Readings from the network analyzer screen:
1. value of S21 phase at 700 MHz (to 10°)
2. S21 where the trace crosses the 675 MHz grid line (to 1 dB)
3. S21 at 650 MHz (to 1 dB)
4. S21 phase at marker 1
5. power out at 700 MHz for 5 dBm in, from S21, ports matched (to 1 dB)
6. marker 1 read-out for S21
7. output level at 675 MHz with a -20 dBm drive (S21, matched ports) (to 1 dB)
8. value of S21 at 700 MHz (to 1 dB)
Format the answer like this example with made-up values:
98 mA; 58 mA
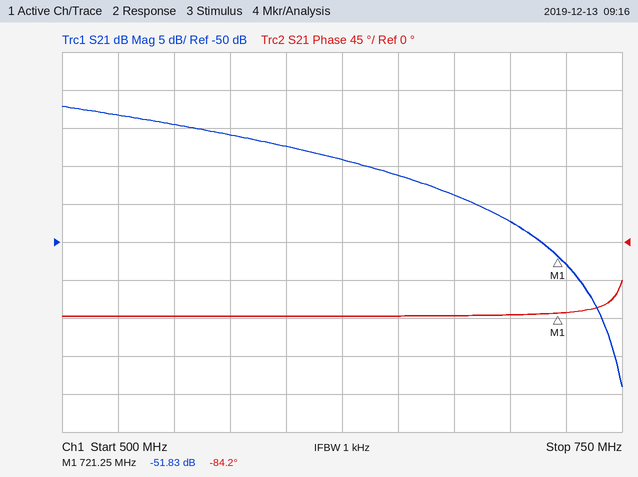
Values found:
-90°; -44 dB; -41 dB; -84.2°; -42 dBm; -51.83 dB; -64 dBm; -47 dB
